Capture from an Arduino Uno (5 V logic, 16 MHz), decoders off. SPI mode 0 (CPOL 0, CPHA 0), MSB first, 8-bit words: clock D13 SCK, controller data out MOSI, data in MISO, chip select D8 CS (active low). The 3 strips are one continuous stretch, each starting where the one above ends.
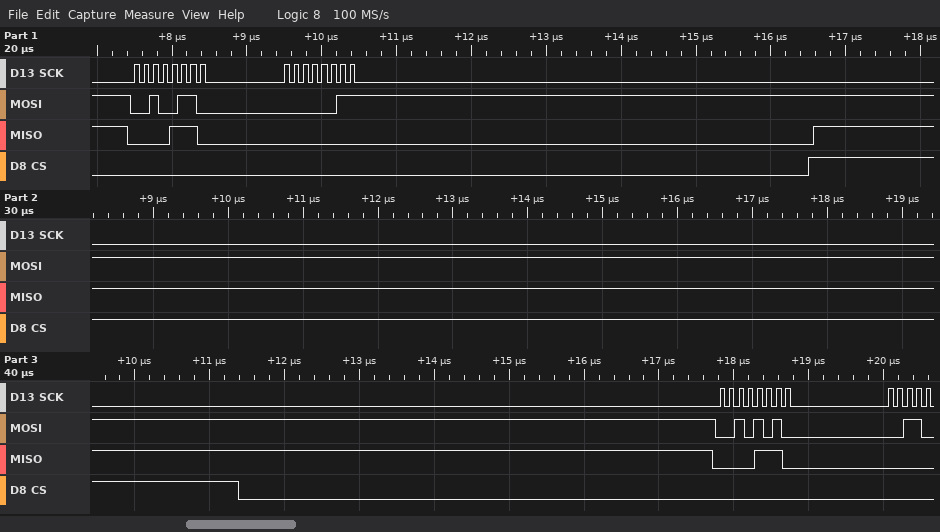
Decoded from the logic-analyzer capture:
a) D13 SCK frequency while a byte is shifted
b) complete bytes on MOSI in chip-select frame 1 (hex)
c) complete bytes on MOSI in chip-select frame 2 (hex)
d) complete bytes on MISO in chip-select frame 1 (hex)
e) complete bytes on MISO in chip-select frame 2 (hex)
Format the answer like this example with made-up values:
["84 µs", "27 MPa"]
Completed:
["8 MHz", "0x26 0x03", "0x2A", "0x0E 0x00", "0x0E"]
